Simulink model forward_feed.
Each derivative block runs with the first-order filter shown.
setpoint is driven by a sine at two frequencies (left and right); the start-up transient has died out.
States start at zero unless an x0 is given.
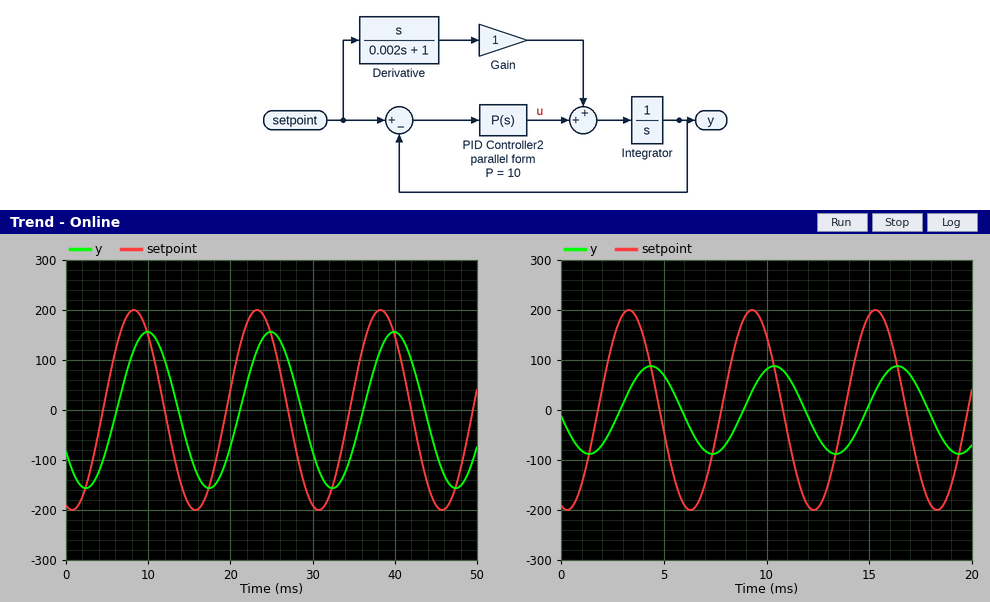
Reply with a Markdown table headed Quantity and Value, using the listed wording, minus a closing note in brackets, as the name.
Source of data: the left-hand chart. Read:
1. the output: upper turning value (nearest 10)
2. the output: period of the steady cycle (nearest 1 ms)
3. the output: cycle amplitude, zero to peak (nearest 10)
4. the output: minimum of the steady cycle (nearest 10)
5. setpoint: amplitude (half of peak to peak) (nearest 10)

| Quantity | Value |
|---|---|
| the output: upper turning value | 160 |
| the output: period of the steady cycle | 15 ms |
| the output: cycle amplitude, zero to peak | 160 |
| the output: minimum of the steady cycle | -160 |
| setpoint: amplitude (half of peak to peak) | 200 |
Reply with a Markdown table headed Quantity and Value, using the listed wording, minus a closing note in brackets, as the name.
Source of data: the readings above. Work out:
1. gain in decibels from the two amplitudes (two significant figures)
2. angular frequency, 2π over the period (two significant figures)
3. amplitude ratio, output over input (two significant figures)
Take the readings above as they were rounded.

| Quantity | Value |
|---|---|
| gain in decibels from the two amplitudes | -1.9 dB |
| angular frequency, 2π over the period | 0.42 rad/ms |
| amplitude ratio, output over input | 0.80 |
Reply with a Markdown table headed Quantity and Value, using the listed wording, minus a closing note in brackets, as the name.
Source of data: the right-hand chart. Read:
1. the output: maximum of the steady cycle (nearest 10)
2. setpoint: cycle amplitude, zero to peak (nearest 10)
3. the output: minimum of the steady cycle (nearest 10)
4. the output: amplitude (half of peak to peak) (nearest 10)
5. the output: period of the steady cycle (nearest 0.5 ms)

| Quantity | Value |
|---|---|
| the output: maximum of the steady cycle | 90 |
| setpoint: cycle amplitude, zero to peak | 200 |
| the output: minimum of the steady cycle | -90 |
| the output: amplitude (half of peak to peak) | 90 |
| the output: period of the steady cycle | 6.0 ms |
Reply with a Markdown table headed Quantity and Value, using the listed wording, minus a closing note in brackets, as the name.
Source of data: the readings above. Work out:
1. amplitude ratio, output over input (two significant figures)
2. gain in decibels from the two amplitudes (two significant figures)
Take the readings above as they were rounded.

| Quantity | Value |
|---|---|
| amplitude ratio, output over input | 0.45 |
| gain in decibels from the two amplitudes | -6.9 dB |
